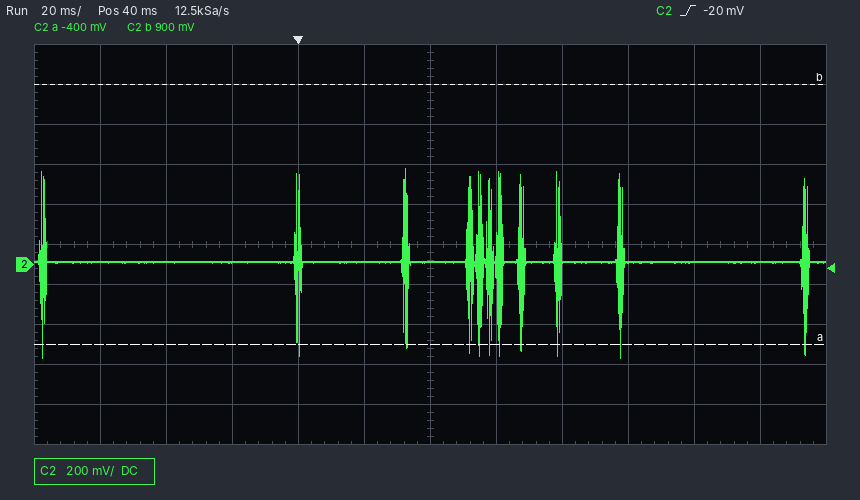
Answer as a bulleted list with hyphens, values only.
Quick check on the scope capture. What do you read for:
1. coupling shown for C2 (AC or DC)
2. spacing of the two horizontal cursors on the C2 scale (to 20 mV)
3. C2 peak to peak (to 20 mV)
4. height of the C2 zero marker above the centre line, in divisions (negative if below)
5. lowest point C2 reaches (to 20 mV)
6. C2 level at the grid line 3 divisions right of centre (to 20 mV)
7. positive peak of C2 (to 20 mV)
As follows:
- DC
- 1.30 V
- 940 mV
- -0.5 div
- -460 mV
- 20 mV
- 480 mV
